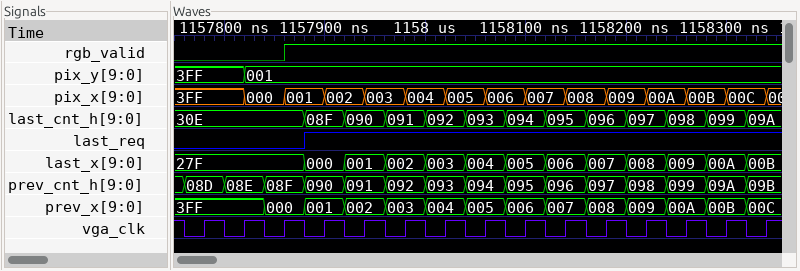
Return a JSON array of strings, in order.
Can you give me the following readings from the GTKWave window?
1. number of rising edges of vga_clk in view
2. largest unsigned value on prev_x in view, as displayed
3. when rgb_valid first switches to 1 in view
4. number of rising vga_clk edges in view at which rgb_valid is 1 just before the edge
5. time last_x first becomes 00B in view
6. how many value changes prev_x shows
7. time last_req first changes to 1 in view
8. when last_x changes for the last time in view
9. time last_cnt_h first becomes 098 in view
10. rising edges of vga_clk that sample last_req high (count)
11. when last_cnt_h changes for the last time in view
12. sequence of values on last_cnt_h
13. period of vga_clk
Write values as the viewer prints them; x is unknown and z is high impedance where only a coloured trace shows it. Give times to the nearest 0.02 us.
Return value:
["15", "3FF", "1157.86 us", "12", "1158.32 us", "13", "1157.88 us", "1158.32 us", "1158.24 us", "12", "1158.32 us", "30E, 08F, 090, 091, 092, 093, 094, 095, 096, 097, 098, 099, 09A", "0.04 us"]
